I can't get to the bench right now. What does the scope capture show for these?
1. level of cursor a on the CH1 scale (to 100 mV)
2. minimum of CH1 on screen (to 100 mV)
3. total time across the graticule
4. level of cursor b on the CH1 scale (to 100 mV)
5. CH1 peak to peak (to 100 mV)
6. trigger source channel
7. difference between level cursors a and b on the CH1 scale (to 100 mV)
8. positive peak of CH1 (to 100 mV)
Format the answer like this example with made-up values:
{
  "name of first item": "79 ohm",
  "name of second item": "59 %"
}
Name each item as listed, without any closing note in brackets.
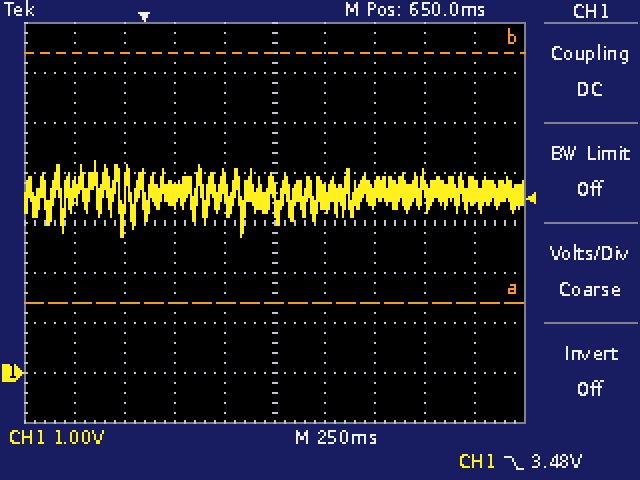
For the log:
{
  "level of cursor a on the CH1 scale": "1.4 V",
  "minimum of CH1 on screen": "2.7 V",
  "total time across the graticule": "2.5 s",
  "level of cursor b on the CH1 scale": "6.4 V",
  "CH1 peak to peak": "1.5 V",
  "trigger source channel": "CH1",
  "difference between level cursors a and b on the CH1 scale": "5.0 V",
  "positive peak of CH1": "4.2 V"
}
